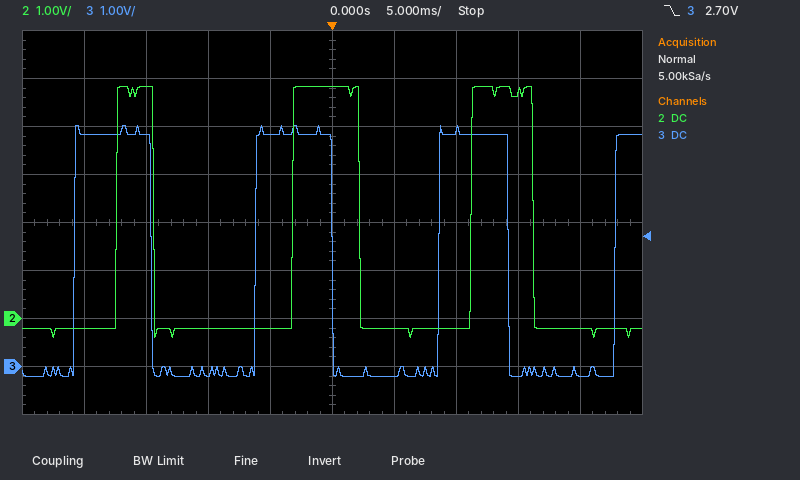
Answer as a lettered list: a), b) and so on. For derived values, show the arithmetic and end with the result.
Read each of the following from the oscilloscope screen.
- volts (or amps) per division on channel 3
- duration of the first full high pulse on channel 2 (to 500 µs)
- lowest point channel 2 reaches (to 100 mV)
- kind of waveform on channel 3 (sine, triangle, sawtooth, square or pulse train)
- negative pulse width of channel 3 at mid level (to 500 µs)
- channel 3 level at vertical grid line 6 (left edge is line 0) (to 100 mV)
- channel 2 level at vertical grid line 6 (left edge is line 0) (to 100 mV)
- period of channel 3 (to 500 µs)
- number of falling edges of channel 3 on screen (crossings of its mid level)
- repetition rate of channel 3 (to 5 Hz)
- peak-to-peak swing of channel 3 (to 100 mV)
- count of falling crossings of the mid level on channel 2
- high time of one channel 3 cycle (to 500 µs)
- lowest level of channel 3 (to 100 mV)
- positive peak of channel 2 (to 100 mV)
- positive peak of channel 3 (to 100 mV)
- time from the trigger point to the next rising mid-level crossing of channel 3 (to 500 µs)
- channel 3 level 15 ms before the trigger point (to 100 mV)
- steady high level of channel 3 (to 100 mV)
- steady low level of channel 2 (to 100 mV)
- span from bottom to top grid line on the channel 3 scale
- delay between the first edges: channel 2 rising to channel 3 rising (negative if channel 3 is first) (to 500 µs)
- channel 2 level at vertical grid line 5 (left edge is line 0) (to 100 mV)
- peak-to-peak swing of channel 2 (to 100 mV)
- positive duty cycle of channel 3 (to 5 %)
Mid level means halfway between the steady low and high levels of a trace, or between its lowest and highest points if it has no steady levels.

a) 1 V
b) 3.0 ms
c) -400 mV
d) pulse train
e) 8.5 ms
f) -200 mV
g) -200 mV
h) 14.5 ms
i) 3
j) 1 / 14.5 ms ≈ 69.0 Hz, so 70 Hz to the nearest 5 Hz
k) 5.0 V − (-200 mV) = 5.2 V
l) 3
m) 6.0 ms
n) -200 mV
o) 4.8 V
p) 5.0 V
q) 8.5 ms
r) 4.8 V
s) 4.8 V
t) -200 mV
u) 8 V
v) -3.5 ms
w) 4.8 V
x) 4.8 V − (-400 mV) = 5.2 V
y) 6.0 ms / 14.5 ms ≈ 41.4 %, so 40 % to the nearest 5 %
